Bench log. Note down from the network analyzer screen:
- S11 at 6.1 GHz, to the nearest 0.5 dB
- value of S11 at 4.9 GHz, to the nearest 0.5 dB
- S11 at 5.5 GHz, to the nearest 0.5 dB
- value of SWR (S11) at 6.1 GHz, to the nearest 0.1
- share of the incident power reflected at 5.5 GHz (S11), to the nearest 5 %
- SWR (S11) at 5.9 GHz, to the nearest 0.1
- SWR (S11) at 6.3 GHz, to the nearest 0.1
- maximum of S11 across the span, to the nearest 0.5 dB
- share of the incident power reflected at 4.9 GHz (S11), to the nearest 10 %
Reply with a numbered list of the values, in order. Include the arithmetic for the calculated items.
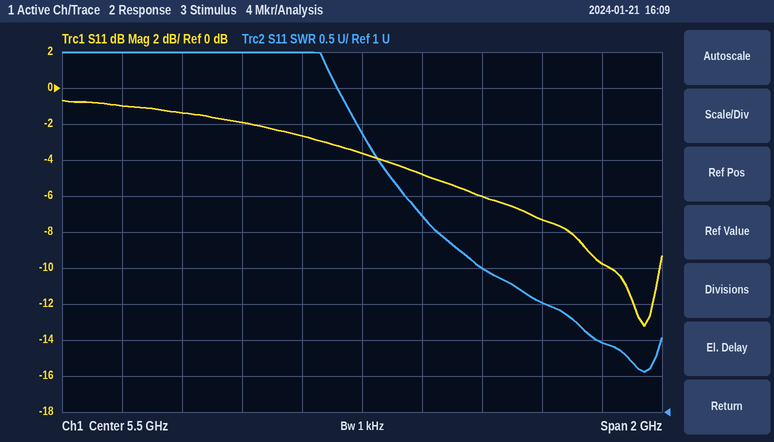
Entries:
1. -7.5 dB
2. -1.5 dB
3. -3.5 dB
4. 2.5
5. 10^(-3.5/10) ≈ 45 %
6. 3.0
7. 2.0
8. -0.5 dB
9. 10^(-1.5/10) ≈ 70.8 %, so 70 % to the nearest 10 %
